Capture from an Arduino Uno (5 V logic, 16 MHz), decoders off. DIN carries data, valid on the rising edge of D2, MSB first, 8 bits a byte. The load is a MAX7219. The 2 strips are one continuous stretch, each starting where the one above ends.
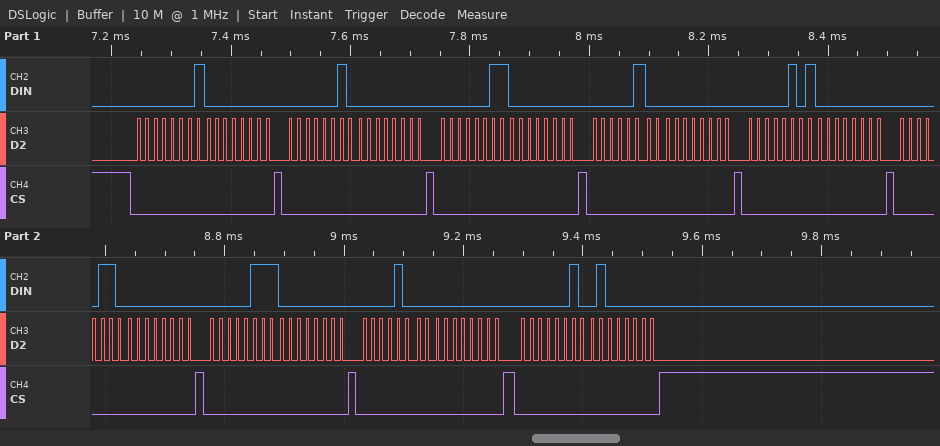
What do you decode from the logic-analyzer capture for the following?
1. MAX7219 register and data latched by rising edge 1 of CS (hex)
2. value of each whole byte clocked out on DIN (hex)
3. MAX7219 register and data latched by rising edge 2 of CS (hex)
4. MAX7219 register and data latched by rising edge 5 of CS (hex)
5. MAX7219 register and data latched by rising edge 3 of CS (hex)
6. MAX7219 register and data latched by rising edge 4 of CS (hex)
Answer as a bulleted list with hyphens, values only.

- register 0x1, data 0x00
- 01 00 02 00 03 00 04 00 05 00 06 00 07 00 08 00 02 40
- register 0x2, data 0x00
- register 0x5, data 0x00
- register 0x3, data 0x00
- register 0x4, data 0x00
